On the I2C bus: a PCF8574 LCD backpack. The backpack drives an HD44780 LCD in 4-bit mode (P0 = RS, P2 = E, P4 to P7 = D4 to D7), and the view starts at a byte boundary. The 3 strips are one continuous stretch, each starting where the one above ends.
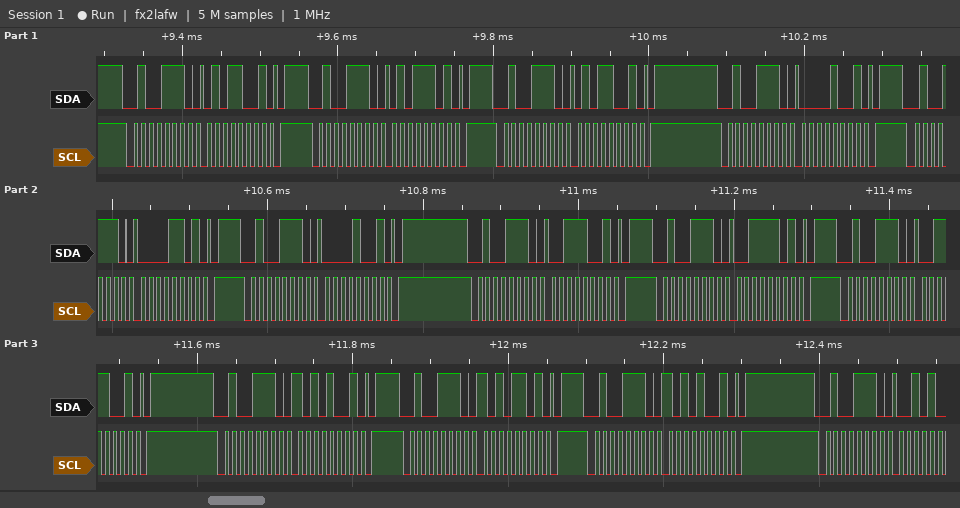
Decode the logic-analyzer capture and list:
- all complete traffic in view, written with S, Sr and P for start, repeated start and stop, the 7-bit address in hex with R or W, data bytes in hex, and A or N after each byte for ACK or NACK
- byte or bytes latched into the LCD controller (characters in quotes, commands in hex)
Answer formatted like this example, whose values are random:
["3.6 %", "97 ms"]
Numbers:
["S 27W A 59 A P S 27W A 5D A P S 27W A 59 A P S 27W A 09 A P S 27W A 0D A P S 27W A 09 A P S 27W A 39 A P S 27W A 3D A P S 27W A 39 A P S 27W A A9 A P S 27W A AD A P S 27W A A9 A P S 27W A", "'P' ':'"]
